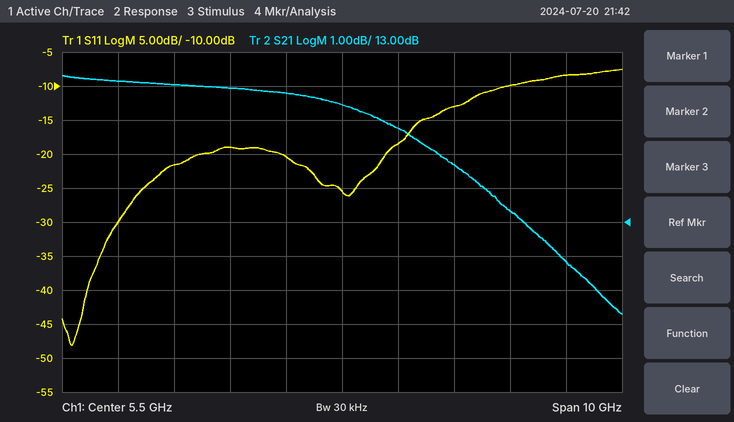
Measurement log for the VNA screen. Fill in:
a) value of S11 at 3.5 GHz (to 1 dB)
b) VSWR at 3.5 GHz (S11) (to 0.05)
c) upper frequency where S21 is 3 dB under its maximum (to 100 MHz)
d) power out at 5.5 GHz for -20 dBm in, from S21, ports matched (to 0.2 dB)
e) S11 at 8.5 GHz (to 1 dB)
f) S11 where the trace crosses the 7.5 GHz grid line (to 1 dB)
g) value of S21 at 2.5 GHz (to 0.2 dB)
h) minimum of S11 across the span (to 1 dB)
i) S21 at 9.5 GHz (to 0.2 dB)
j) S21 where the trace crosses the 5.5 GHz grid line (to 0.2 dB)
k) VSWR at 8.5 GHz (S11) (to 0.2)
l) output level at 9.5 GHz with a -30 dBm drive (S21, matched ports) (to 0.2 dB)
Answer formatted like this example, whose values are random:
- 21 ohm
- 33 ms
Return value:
- -19 dB
- 1.25
- 7.8 GHz
- -3.6 dBm
- -10 dB
- -13 dB
- 17.0 dB
- -48 dB
- 11.8 dB
- 16.4 dB
- 2.0
- -18.2 dBm
